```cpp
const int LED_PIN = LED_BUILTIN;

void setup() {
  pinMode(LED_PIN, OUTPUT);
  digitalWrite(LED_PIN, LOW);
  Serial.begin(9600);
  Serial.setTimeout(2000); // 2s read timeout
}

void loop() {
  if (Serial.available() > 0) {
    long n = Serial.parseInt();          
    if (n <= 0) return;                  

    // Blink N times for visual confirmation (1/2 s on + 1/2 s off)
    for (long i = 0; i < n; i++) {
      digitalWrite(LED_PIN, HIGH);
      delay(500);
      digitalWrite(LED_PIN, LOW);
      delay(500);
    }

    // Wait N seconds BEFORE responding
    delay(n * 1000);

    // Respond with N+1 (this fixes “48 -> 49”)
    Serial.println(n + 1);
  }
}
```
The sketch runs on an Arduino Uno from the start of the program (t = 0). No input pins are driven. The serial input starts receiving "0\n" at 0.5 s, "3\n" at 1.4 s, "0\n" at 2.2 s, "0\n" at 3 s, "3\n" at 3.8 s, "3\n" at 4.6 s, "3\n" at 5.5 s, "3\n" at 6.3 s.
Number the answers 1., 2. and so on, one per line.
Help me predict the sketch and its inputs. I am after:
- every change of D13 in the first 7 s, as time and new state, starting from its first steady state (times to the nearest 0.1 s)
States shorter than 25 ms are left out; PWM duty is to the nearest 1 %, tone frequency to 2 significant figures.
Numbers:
1. 0 s low; 1.4 s high; 1.9 s low; 2.4 s high; 2.9 s low; 3.4 s high; 3.9 s low
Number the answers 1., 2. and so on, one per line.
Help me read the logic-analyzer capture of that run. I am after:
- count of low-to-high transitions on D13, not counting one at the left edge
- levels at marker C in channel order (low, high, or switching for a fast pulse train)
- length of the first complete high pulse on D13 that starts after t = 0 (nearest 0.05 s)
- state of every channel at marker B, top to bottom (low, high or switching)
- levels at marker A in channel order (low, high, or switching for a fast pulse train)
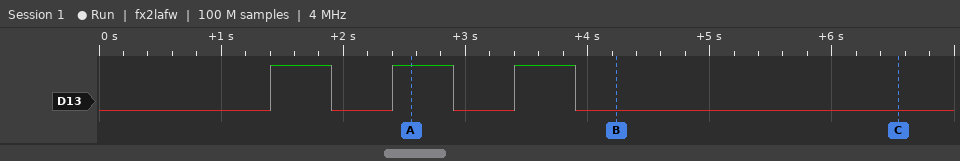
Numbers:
1. 3
2. D13 low
3. 0.50 s
4. D13 low
5. D13 high
